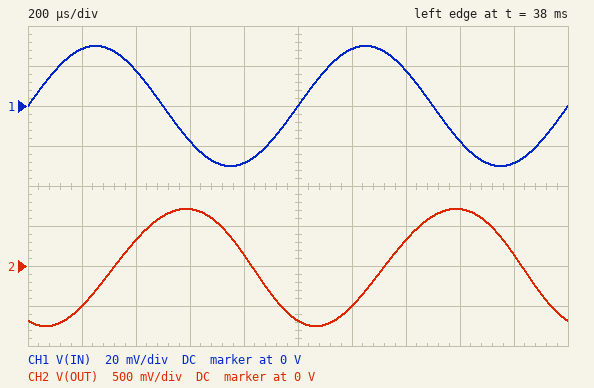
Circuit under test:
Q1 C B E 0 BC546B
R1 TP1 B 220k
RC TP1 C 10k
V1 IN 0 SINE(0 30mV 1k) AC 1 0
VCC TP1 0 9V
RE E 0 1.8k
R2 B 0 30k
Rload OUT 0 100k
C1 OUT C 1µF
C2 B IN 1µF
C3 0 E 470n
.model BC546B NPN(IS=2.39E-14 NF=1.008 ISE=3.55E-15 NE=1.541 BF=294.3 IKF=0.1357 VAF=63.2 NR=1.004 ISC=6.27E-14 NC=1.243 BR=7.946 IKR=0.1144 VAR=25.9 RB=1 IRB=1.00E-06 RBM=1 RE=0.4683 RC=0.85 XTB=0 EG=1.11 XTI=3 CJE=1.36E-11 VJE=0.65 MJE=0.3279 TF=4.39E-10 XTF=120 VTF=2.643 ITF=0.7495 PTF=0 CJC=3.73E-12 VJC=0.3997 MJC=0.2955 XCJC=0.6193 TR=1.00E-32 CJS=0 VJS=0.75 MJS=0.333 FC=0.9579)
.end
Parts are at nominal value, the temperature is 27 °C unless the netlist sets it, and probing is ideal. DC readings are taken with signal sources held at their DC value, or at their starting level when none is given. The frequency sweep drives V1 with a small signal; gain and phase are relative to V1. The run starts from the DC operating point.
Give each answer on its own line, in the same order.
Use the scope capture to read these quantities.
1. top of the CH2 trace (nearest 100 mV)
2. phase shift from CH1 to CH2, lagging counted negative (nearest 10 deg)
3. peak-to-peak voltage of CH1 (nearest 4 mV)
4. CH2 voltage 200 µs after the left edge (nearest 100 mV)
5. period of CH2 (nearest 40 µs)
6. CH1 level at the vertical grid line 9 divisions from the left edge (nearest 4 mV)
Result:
700 mV
-120 deg
60 mV
-500 mV
1.00 ms
-28 mV
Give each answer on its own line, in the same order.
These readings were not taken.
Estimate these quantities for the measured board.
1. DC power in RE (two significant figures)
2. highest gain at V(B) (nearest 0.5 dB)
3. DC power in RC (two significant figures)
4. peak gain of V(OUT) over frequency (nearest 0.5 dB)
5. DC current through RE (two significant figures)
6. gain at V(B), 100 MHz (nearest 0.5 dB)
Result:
120 µW
0 dB
640 µW
38.5 dB
250 µA
0 dB
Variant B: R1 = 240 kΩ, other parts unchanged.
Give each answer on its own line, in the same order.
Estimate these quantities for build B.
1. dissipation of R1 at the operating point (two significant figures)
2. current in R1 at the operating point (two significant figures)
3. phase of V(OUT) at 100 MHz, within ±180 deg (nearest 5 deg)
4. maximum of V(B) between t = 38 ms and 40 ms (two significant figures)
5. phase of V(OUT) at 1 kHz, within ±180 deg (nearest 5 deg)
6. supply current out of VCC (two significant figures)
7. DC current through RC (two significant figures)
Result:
270 µW
33 µA
85 deg
1.0 V
-120 deg
250 µA
210 µA
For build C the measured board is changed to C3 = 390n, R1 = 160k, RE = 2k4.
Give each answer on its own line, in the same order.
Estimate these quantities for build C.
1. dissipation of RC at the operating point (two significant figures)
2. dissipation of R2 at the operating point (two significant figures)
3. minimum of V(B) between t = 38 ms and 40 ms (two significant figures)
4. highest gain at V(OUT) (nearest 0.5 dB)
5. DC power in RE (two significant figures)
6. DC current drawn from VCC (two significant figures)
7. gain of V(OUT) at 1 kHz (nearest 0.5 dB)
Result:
1.1 mW
65 µW
1.4 V
40.5 dB
260 µW
370 µA
26.5 dB
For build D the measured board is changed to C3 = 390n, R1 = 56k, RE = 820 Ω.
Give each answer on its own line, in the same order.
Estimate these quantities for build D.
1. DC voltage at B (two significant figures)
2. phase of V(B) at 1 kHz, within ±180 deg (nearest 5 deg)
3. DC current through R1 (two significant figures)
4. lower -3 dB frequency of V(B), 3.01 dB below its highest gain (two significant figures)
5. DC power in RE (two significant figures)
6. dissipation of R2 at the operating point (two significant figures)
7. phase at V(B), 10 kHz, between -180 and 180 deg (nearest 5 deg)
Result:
1.4 V
10 deg
140 µA
310 Hz
680 µW
65 µW
5 deg
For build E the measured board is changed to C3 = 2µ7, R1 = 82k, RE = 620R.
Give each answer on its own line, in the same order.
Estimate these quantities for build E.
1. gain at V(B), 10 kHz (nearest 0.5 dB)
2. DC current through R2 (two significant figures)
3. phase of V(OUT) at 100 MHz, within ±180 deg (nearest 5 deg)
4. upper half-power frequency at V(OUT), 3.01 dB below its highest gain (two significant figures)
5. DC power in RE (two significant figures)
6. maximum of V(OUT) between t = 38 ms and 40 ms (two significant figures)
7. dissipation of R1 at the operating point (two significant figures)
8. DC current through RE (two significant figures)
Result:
0 dB
40 µA
70 deg
61 MHz
500 µW
2.2 V
740 µW
900 µA
